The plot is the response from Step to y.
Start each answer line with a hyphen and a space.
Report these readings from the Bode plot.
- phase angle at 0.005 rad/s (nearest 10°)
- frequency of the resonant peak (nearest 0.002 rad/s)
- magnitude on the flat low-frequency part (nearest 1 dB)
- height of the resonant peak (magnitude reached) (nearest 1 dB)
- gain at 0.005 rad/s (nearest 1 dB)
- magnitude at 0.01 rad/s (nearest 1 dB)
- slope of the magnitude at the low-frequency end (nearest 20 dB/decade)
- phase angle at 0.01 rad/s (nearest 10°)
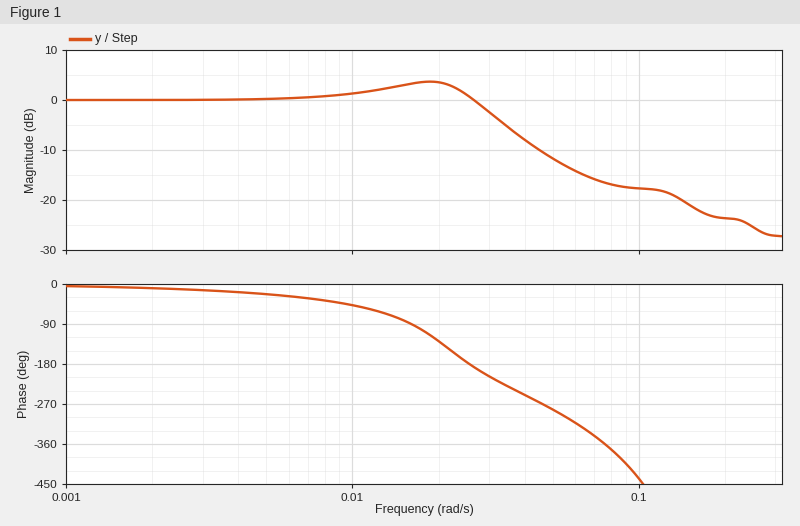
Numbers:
- -20°
- 0.018 rad/s
- 0 dB
- 4 dB
- 0 dB
- 1 dB
- 0 dB/decade
- -50°
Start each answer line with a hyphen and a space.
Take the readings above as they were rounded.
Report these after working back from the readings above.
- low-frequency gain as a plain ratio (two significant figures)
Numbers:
- 1.0
